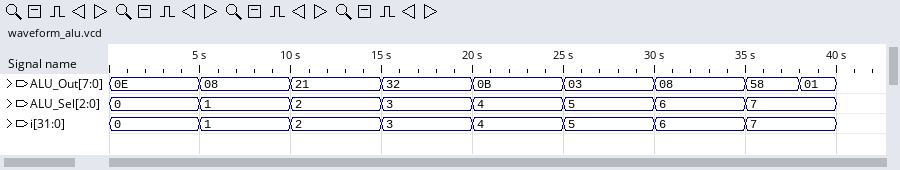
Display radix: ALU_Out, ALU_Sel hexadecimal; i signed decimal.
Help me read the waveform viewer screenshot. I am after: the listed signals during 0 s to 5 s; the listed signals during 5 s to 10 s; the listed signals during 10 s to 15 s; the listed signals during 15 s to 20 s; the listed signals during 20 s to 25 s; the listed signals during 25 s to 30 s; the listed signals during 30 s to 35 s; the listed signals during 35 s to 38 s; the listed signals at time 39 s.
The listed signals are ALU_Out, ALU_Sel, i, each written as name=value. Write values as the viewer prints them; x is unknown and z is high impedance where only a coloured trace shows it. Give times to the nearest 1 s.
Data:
ALU_Out=0E, ALU_Sel=0, i=0
ALU_Out=08, ALU_Sel=1, i=1
ALU_Out=21, ALU_Sel=2, i=2
ALU_Out=32, ALU_Sel=3, i=3
ALU_Out=0B, ALU_Sel=4, i=4
ALU_Out=03, ALU_Sel=5, i=5
ALU_Out=08, ALU_Sel=6, i=6
ALU_Out=58, ALU_Sel=7, i=7
ALU_Out=01, ALU_Sel=7, i=7
